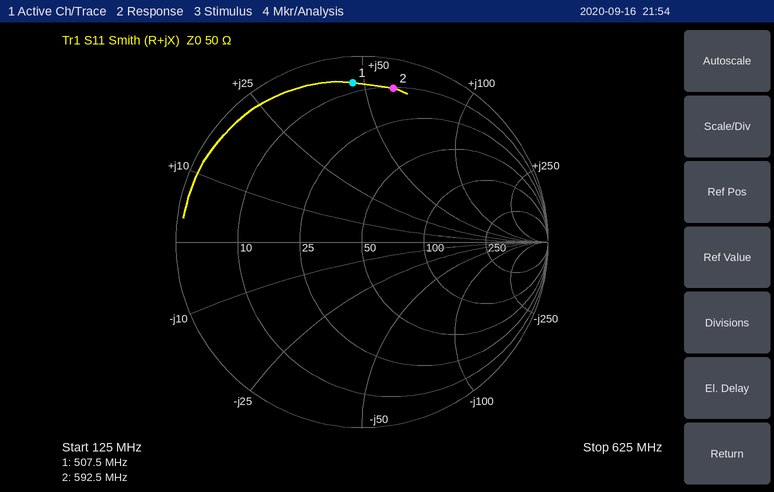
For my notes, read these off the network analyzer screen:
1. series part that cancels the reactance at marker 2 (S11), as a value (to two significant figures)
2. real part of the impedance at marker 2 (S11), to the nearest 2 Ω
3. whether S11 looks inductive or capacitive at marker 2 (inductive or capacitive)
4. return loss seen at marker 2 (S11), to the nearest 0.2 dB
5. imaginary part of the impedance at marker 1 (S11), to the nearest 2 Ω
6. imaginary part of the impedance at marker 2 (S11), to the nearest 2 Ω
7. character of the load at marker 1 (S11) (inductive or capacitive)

4.5 pF
10 Ω
inductive
1.4 dB
+46 Ω
+60 Ω
inductive
